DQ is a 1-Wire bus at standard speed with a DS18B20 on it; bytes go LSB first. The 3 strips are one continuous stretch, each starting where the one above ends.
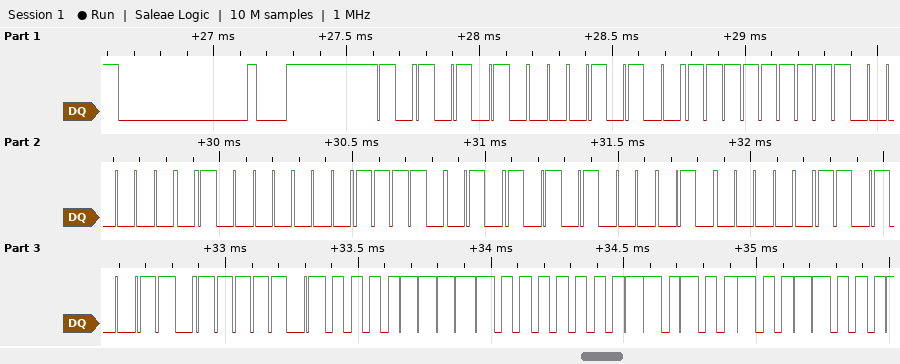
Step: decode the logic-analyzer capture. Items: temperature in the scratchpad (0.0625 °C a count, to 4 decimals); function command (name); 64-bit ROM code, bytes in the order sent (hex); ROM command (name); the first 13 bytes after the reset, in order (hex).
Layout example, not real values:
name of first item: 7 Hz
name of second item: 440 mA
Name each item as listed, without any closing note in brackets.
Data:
temperature in the scratchpad: 31.0000 °C
function command: Read Scratchpad
64-bit ROM code, bytes in the order sent: 28 FF 01 01 4F 15 02 CB
ROM command: Match ROM
the first 13 bytes after the reset, in order: 55 28 FF 01 01 4F 15 02 CB BE F0 01 4B
